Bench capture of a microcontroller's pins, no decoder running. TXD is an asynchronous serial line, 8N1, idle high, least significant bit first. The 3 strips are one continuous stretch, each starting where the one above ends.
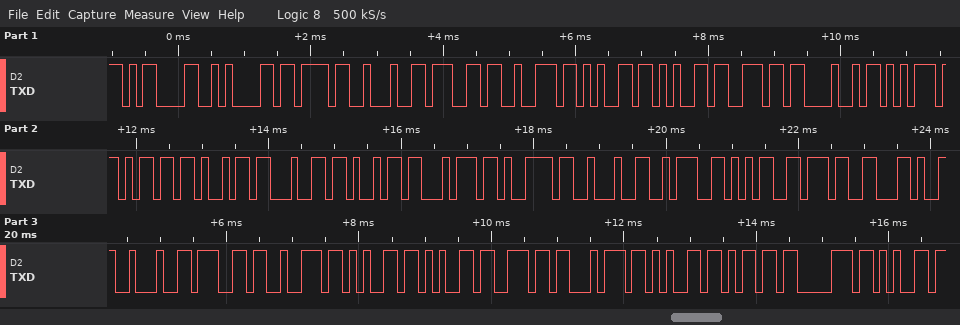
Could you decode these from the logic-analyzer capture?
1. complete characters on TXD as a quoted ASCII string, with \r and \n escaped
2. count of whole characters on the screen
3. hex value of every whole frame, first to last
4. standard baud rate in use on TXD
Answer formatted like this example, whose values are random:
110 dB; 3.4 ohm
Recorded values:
"\r\n{\"greenHumidity\":57,\"greentempe"; 33; 0D 0A 7B 22 67 72 65 65 6E 48 75 6D 69 64 69 74 79 22 3A 35 37 2C 22 67 72 65 65 6E 74 65 6D 70 65; 9600 baud
